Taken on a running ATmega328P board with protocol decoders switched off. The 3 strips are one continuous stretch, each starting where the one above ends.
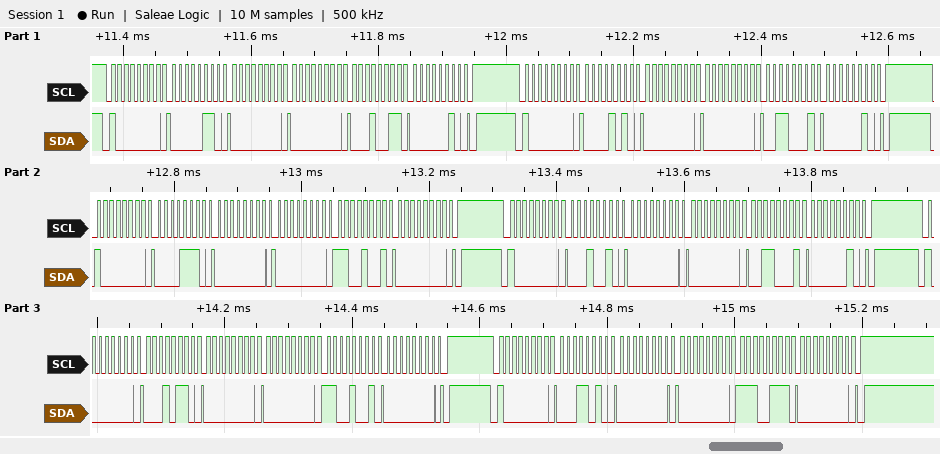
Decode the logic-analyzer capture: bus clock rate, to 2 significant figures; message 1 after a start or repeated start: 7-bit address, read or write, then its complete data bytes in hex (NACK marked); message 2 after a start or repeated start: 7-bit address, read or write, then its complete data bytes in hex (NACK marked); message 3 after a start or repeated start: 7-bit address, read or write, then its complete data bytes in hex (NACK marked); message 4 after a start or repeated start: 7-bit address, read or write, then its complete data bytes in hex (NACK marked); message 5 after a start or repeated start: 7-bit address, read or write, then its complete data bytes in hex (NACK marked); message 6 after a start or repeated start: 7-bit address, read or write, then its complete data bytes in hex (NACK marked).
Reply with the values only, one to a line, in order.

100 kHz
0x40 write: 06 00 00 13 02
0x40 write: 0A 00 00 31 02
0x40 write: 0E 00 00 C9 00
0x40 write: 12 00 00 31 02
0x40 write: 16 00 00 C9 00
0x40 write: 1A 00 00 E7 00
